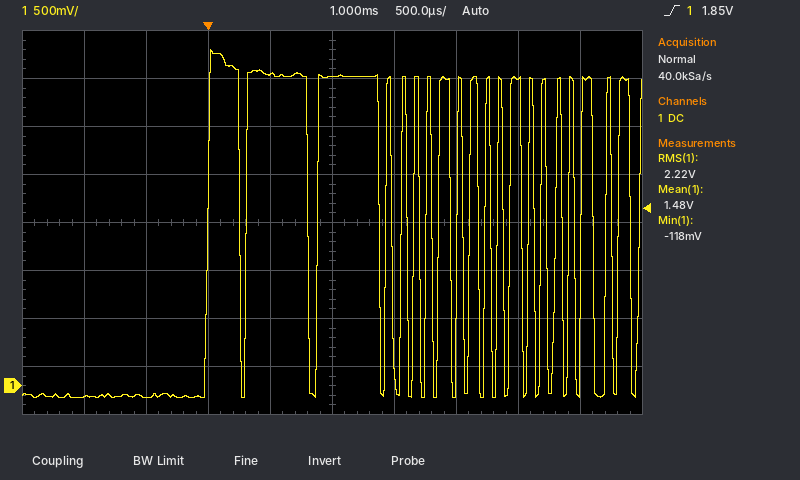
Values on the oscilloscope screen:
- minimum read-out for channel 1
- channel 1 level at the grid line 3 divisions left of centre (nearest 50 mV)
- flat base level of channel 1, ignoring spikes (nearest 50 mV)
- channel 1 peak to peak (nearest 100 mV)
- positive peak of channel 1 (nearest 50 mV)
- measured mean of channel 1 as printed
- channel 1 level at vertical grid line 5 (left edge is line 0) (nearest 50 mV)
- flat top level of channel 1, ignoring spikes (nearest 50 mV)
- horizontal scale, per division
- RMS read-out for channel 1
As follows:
-118 mV
-100 mV
-100 mV
3.60 V
3.50 V
1.48 V
3.20 V
3.20 V
500 µs
2.22 V
